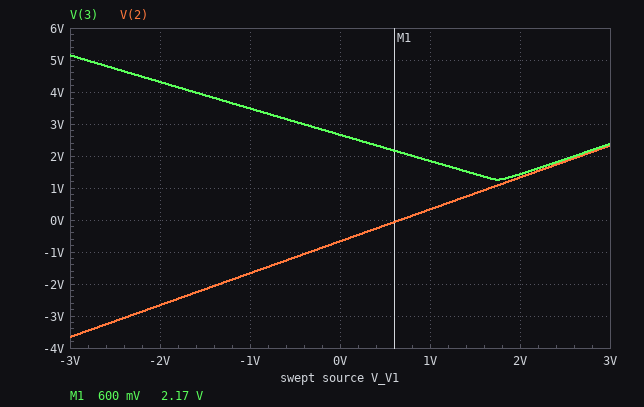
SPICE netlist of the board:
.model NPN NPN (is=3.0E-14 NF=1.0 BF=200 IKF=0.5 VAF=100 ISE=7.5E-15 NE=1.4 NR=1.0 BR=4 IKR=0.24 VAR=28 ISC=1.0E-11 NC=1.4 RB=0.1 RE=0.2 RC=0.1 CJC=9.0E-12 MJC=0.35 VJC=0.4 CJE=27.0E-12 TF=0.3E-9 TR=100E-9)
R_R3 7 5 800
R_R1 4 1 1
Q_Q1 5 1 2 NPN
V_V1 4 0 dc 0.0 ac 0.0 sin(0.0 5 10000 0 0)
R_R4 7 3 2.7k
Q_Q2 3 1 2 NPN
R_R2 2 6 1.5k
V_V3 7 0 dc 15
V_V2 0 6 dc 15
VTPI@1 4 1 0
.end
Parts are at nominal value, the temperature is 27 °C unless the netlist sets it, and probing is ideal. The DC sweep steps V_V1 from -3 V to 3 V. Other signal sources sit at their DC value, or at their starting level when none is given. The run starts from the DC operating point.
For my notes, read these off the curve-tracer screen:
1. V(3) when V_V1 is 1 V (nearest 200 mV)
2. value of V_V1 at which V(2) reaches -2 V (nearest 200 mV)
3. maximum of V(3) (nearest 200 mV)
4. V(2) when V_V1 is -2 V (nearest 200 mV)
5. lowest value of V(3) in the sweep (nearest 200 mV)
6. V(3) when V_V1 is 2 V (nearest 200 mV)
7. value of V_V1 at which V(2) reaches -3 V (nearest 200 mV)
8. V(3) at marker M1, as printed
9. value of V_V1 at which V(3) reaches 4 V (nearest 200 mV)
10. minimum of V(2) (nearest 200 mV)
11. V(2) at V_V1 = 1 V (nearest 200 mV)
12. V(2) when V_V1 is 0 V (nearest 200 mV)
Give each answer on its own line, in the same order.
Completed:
1.8 V
-1.4 V
5.2 V
-2.6 V
1.2 V
1.4 V
-2.4 V
2.17 V
-1.6 V
-3.6 V
400 mV
-600 mV
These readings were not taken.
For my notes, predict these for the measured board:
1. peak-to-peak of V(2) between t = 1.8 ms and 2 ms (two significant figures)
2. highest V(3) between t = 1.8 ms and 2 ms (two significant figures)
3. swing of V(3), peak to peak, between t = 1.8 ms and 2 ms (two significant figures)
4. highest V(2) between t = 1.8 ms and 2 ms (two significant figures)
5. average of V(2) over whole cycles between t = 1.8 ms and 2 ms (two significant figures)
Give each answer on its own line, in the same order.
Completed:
10 V
6.8 V
5.6 V
4.3 V
-670 mV
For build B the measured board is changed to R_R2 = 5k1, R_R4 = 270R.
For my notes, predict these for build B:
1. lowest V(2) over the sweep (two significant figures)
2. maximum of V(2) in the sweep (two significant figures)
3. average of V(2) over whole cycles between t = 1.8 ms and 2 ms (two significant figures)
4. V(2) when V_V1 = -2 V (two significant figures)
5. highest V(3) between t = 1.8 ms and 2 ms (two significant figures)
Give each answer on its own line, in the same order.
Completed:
-3.6 V
2.4 V
-630 mV
-2.6 V
15 V
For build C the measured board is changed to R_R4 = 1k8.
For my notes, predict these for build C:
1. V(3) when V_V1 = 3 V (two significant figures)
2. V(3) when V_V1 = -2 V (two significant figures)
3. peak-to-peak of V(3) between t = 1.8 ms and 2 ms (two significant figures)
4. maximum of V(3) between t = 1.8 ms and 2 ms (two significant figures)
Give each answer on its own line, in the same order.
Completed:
4.9 V
7.8 V
5.4 V
9.5 V
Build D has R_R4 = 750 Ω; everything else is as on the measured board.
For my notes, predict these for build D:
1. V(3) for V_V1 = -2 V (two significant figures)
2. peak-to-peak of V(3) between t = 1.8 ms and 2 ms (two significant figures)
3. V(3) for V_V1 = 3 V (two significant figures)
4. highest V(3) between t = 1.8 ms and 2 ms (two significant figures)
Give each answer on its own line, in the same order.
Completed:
12 V
2.5 V
11 V
13 V
